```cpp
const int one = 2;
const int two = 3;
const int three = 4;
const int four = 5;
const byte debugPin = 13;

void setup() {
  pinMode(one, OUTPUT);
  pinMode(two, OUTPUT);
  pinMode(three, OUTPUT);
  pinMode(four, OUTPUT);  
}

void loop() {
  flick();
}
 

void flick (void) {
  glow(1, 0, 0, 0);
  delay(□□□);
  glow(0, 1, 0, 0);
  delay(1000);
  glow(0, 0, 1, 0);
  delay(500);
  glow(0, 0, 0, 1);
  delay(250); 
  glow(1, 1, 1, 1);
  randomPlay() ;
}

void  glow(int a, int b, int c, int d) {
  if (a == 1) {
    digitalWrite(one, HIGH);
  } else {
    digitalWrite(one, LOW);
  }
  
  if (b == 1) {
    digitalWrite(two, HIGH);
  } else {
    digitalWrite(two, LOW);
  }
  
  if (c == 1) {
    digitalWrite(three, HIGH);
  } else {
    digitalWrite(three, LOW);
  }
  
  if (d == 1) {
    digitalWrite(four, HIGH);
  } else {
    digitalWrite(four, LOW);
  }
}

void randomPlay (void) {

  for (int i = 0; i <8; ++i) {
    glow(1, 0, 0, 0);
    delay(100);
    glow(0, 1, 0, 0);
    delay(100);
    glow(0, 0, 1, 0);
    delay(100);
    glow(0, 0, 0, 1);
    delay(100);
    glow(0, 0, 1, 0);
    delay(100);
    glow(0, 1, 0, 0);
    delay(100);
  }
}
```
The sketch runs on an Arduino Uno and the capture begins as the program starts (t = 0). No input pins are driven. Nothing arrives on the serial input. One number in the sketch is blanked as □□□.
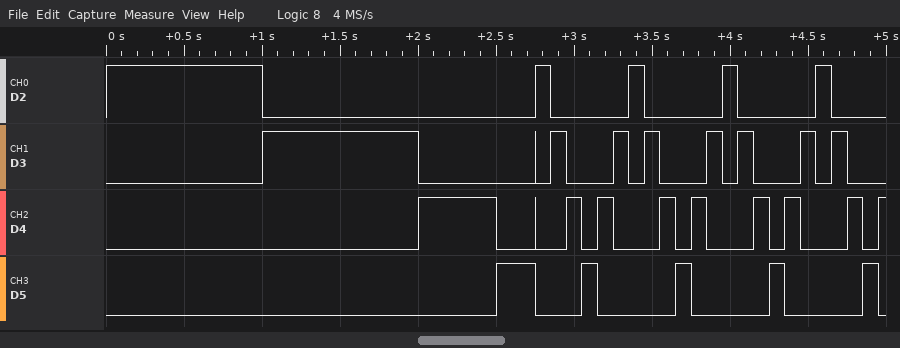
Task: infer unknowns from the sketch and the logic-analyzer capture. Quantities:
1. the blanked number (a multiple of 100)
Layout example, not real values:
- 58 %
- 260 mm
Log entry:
- 1000
